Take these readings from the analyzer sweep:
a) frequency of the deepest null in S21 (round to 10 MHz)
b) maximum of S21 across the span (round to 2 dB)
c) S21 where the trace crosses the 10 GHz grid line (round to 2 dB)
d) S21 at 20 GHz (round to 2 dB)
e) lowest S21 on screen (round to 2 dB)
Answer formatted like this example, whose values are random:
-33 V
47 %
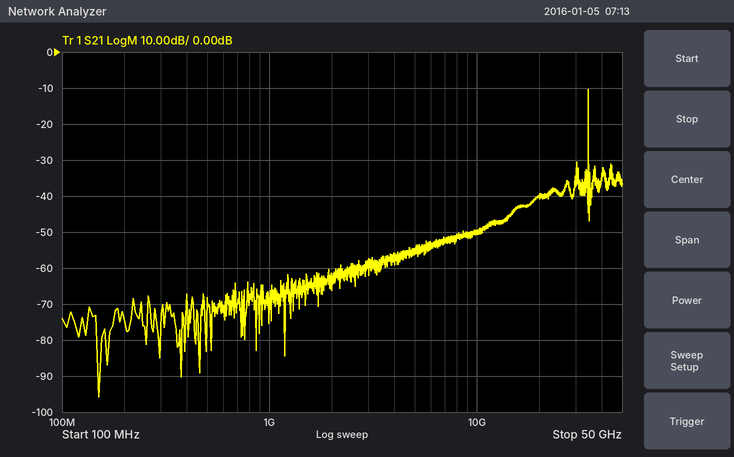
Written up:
150 MHz
-10 dB
-50 dB
-40 dB
-96 dB
